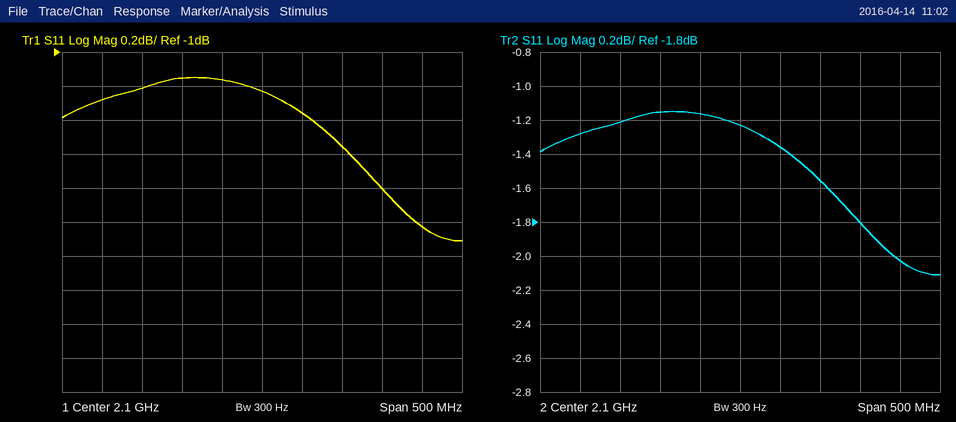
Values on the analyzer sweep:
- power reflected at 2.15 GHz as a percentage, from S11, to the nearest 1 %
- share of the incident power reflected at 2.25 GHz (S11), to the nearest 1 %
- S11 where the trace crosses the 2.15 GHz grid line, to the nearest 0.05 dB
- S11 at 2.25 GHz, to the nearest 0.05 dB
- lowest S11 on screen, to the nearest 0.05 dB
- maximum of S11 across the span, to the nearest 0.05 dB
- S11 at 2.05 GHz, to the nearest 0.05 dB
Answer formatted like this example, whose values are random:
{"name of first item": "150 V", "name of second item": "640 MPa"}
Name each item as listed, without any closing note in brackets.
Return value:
{"power reflected at 2.15 GHz as a percentage, from S11, to the nearest 1 %": "73 %", "share of the incident power reflected at 2.25 GHz (S11), to the nearest 1 %": "66 %", "S11 where the trace crosses the 2.15 GHz grid line, to the nearest 0.05 dB": "-1.35 dB", "S11 at 2.25 GHz, to the nearest 0.05 dB": "-1.80 dB", "lowest S11 on screen, to the nearest 0.05 dB": "-2.10 dB", "maximum of S11 across the span, to the nearest 0.05 dB": "-1.15 dB", "S11 at 2.05 GHz, to the nearest 0.05 dB": "-1.15 dB"}
